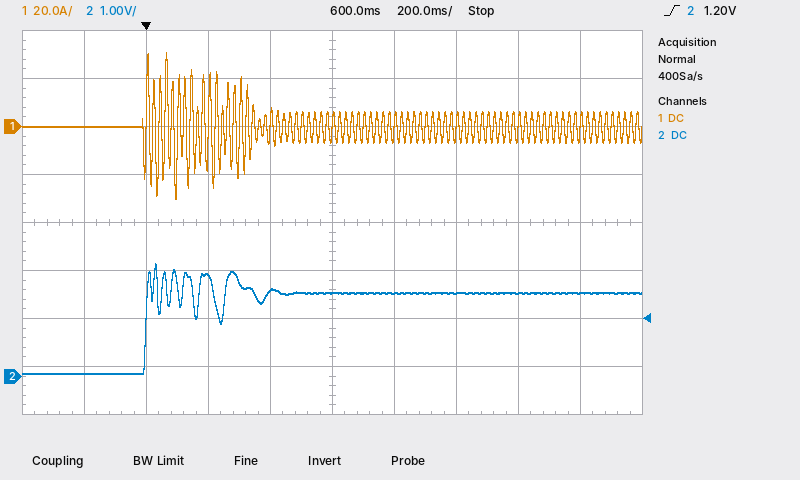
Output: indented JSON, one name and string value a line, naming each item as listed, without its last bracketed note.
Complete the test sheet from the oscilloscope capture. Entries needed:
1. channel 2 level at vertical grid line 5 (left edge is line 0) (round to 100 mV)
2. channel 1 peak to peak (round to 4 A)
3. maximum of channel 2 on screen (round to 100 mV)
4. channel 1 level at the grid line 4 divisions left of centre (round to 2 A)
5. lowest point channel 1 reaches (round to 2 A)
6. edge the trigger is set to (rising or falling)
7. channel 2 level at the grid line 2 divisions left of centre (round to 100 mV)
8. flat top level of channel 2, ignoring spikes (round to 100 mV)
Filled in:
{
  "channel 2 level at vertical grid line 5 (left edge is line 0)": "1.7 V",
  "channel 1 peak to peak": "60 A",
  "maximum of channel 2 on screen": "2.3 V",
  "channel 1 level at the grid line 4 divisions left of centre": "0 A",
  "lowest point channel 1 reaches": "-30 A",
  "edge the trigger is set to": "rising",
  "channel 2 level at the grid line 2 divisions left of centre": "2.1 V",
  "flat top level of channel 2, ignoring spikes": "1.7 V"
}
